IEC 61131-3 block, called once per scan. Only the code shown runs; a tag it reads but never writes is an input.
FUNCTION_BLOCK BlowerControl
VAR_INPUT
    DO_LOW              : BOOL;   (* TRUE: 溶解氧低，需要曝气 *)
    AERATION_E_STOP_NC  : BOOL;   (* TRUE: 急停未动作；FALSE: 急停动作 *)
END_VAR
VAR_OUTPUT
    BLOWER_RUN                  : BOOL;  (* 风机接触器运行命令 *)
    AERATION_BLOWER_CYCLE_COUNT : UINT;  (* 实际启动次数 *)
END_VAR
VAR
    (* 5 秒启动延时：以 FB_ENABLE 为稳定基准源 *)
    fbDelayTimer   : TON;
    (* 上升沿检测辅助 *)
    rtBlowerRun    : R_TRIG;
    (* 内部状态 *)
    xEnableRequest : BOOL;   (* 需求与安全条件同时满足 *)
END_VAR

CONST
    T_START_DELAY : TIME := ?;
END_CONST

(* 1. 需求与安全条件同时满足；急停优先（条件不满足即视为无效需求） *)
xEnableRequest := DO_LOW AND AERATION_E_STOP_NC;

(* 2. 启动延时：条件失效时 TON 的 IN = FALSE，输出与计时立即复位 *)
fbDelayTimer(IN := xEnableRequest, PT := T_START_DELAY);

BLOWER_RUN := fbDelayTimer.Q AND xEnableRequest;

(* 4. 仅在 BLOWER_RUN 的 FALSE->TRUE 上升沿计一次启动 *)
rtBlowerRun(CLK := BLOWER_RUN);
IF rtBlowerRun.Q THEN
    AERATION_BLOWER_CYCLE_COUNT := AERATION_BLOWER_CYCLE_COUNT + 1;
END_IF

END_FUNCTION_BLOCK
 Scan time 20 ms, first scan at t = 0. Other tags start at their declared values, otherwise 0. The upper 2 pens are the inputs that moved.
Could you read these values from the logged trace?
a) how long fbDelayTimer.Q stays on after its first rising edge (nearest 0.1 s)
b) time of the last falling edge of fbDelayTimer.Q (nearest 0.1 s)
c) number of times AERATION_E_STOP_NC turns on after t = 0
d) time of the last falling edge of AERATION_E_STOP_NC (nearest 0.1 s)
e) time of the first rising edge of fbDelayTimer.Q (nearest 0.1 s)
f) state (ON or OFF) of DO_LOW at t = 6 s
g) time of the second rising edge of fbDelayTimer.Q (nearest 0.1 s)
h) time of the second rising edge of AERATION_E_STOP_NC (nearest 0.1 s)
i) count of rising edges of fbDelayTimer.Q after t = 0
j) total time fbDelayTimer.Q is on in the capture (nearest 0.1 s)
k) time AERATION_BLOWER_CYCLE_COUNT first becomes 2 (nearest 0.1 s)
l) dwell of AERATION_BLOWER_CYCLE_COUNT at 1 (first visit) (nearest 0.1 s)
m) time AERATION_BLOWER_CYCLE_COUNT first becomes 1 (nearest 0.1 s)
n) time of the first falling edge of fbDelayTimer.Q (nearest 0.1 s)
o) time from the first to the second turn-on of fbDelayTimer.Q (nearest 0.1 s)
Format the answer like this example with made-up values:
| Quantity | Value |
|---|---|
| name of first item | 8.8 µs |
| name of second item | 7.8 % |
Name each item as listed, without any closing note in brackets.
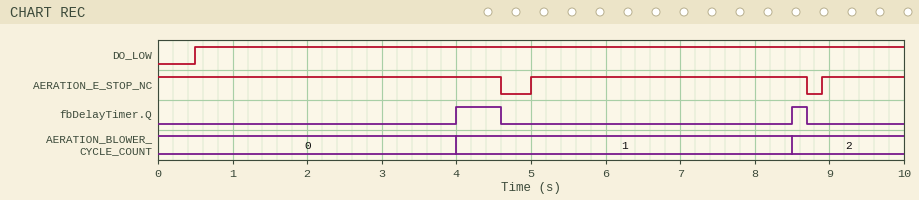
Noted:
| Quantity | Value |
|---|---|
| how long fbDelayTimer.Q stays on after its first rising edge | 0.6 s |
| time of the last falling edge of fbDelayTimer.Q | 8.7 s |
| number of times AERATION_E_STOP_NC turns on after t = 0 | 2 |
| time of the last falling edge of AERATION_E_STOP_NC | 8.7 s |
| time of the first rising edge of fbDelayTimer.Q | 4.0 s |
| state (ON or OFF) of DO_LOW at t = 6 s | ON |
| time of the second rising edge of fbDelayTimer.Q | 8.5 s |
| time of the second rising edge of AERATION_E_STOP_NC | 8.9 s |
| count of rising edges of fbDelayTimer.Q after t = 0 | 2 |
| total time fbDelayTimer.Q is on in the capture | 0.8 s |
| time AERATION_BLOWER_CYCLE_COUNT first becomes 2 | 8.5 s |
| dwell of AERATION_BLOWER_CYCLE_COUNT at 1 (first visit) | 4.5 s |
| time AERATION_BLOWER_CYCLE_COUNT first becomes 1 | 4.0 s |
| time of the first falling edge of fbDelayTimer.Q | 4.6 s |
| time from the first to the second turn-on of fbDelayTimer.Q | 4.5 s |
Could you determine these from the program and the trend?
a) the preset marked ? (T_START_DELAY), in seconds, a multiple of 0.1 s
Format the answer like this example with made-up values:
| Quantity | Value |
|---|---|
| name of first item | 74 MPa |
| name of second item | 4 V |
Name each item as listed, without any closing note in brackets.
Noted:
| Quantity | Value |
|---|---|
| the preset marked ? (T_START_DELAY), in seconds, a multiple of 0.1 s | 3.5 s |
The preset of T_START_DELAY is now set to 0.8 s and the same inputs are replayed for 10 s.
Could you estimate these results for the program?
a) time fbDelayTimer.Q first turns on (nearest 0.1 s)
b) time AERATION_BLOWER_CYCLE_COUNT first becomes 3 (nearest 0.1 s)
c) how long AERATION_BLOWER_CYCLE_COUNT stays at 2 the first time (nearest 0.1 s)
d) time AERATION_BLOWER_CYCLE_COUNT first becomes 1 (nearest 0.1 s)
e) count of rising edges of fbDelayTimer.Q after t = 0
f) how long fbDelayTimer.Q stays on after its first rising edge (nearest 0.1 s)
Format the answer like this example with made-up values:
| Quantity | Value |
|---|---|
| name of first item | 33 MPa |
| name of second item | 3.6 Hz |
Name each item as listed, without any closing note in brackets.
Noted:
| Quantity | Value |
|---|---|
| time fbDelayTimer.Q first turns on | 1.3 s |
| time AERATION_BLOWER_CYCLE_COUNT first becomes 3 | 9.7 s |
| how long AERATION_BLOWER_CYCLE_COUNT stays at 2 the first time | 3.9 s |
| time AERATION_BLOWER_CYCLE_COUNT first becomes 1 | 1.3 s |
| count of rising edges of fbDelayTimer.Q after t = 0 | 3 |
| how long fbDelayTimer.Q stays on after its first rising edge | 3.3 s |
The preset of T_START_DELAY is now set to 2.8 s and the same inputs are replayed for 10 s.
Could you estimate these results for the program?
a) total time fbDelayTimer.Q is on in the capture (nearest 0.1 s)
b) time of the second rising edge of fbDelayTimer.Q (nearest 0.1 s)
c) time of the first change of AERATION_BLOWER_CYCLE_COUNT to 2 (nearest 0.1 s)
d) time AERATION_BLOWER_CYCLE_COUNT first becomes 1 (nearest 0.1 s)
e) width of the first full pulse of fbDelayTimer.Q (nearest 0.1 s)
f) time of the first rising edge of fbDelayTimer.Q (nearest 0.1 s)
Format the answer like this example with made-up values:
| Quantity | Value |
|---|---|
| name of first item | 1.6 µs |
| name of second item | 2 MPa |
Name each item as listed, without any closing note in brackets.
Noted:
| Quantity | Value |
|---|---|
| total time fbDelayTimer.Q is on in the capture | 2.2 s |
| time of the second rising edge of fbDelayTimer.Q | 7.8 s |
| time of the first change of AERATION_BLOWER_CYCLE_COUNT to 2 | 7.8 s |
| time AERATION_BLOWER_CYCLE_COUNT first becomes 1 | 3.3 s |
| width of the first full pulse of fbDelayTimer.Q | 1.3 s |
| time of the first rising edge of fbDelayTimer.Q | 3.3 s |
